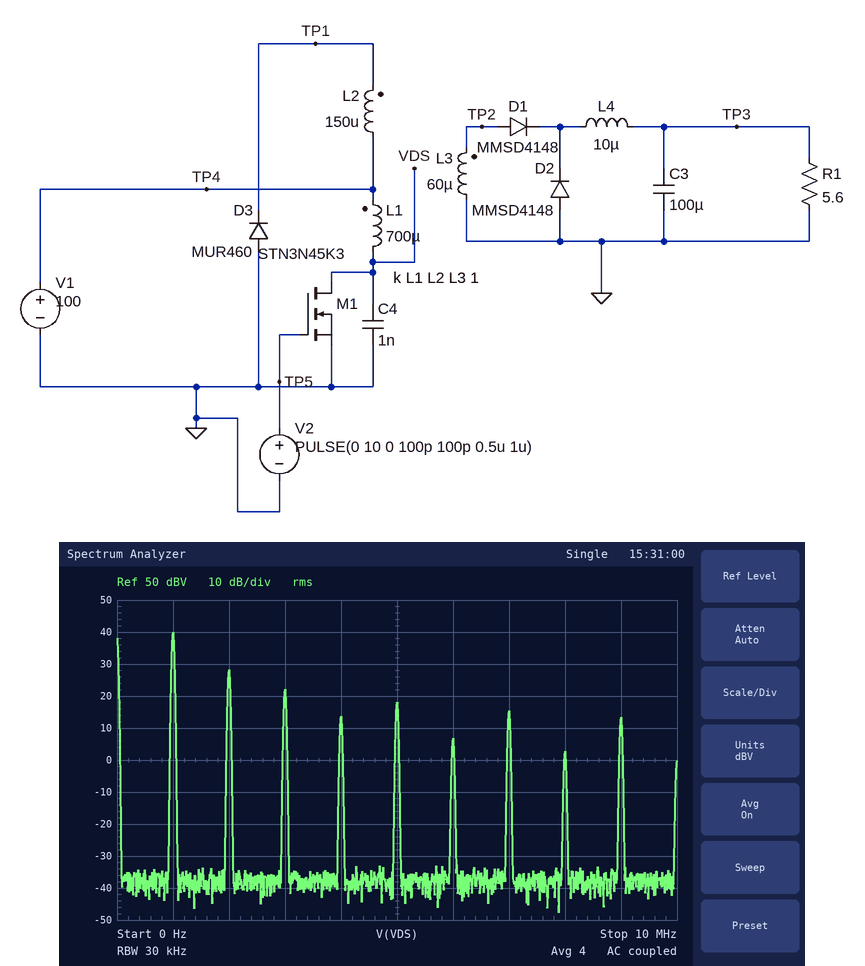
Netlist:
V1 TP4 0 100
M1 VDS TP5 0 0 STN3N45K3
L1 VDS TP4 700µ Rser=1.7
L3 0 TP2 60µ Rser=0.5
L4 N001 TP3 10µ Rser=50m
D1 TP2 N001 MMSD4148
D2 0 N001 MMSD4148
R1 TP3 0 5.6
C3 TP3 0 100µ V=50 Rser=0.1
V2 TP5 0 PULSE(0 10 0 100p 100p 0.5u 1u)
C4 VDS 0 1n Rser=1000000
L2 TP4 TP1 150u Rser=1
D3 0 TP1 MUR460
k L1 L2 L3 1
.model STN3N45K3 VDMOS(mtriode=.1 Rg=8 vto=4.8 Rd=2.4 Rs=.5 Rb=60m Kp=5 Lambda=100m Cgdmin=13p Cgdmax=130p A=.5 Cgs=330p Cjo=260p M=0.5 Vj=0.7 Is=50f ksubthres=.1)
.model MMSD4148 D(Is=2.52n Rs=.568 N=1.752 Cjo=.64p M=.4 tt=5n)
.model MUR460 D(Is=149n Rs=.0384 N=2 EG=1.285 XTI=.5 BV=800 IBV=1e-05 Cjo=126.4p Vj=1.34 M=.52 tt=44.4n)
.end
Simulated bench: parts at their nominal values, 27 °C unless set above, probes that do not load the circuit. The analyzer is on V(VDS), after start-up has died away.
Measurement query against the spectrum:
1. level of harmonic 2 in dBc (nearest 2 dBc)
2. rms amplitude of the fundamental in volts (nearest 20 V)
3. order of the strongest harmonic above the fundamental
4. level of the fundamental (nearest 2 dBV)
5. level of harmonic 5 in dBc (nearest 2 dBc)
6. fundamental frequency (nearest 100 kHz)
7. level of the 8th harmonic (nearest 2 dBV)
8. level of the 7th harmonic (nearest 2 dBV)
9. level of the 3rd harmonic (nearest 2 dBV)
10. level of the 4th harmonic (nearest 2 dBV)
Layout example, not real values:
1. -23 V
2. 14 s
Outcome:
1. -12 dBc
2. 100 V
3. 2
4. 40 dBV
5. -22 dBc
6. 1.0 MHz
7. 2 dBV
8. 16 dBV
9. 22 dBV
10. 14 dBV
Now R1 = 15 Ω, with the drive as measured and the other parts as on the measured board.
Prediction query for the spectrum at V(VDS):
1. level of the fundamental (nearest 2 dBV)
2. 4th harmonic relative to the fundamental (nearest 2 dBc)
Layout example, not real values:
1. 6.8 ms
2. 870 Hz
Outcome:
1. 40 dBV
2. -24 dBc
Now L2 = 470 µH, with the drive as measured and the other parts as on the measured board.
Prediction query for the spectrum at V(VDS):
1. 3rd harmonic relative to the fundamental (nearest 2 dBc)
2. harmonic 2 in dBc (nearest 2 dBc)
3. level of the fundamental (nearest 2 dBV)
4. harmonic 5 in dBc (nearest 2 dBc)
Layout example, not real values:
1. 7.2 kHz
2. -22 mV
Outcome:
1. -12 dBc
2. -16 dBc
3. 40 dBV
4. -18 dBc
